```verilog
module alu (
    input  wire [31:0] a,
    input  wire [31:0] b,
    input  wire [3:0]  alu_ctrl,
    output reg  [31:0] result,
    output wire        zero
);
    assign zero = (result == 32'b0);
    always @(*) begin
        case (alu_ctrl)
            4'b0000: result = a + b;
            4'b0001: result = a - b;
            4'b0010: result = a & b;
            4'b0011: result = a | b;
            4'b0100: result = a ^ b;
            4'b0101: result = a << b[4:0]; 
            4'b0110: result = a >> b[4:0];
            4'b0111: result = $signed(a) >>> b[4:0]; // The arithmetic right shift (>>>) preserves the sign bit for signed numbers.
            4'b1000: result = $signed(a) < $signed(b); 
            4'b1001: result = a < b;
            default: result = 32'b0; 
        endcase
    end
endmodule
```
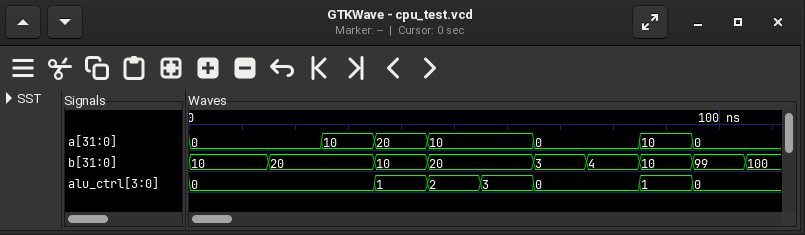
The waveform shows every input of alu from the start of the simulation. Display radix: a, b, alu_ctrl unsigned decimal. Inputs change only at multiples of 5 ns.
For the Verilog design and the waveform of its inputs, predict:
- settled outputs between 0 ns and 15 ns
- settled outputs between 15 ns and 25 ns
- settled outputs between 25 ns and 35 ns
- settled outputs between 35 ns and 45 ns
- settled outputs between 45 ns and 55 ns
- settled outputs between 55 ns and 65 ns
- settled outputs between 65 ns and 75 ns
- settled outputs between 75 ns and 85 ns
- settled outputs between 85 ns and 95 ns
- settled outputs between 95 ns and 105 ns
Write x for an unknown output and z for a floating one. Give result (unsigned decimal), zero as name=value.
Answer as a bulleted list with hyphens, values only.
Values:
- result=10, zero=0
- result=20, zero=0
- result=30, zero=0
- result=10, zero=0
- result=0, zero=1
- result=30, zero=0
- result=3, zero=0
- result=4, zero=0
- result=0, zero=1
- result=99, zero=0
